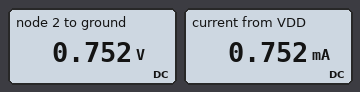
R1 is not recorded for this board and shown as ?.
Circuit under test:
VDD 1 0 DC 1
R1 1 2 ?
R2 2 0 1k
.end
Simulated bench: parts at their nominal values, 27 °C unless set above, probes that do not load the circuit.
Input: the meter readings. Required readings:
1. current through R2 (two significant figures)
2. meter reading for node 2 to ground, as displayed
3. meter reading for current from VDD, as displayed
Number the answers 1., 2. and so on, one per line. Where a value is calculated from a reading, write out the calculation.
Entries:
1. (752 mV) / 1 kΩ = 750 µA
2. 0.752 V
3. 0.752 mA
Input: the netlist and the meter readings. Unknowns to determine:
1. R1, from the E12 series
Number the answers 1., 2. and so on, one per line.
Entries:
1. 330 Ω
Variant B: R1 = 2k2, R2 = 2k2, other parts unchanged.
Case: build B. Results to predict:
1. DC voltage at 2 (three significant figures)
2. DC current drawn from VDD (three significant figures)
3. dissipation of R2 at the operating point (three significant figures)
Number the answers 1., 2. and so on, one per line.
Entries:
1. 500 mV
2. 227 µA
3. 114 µW
